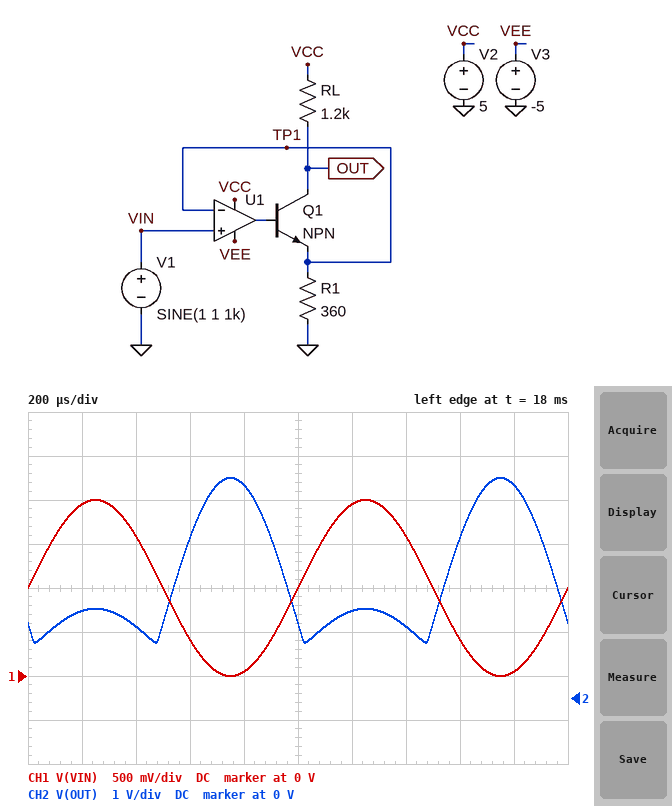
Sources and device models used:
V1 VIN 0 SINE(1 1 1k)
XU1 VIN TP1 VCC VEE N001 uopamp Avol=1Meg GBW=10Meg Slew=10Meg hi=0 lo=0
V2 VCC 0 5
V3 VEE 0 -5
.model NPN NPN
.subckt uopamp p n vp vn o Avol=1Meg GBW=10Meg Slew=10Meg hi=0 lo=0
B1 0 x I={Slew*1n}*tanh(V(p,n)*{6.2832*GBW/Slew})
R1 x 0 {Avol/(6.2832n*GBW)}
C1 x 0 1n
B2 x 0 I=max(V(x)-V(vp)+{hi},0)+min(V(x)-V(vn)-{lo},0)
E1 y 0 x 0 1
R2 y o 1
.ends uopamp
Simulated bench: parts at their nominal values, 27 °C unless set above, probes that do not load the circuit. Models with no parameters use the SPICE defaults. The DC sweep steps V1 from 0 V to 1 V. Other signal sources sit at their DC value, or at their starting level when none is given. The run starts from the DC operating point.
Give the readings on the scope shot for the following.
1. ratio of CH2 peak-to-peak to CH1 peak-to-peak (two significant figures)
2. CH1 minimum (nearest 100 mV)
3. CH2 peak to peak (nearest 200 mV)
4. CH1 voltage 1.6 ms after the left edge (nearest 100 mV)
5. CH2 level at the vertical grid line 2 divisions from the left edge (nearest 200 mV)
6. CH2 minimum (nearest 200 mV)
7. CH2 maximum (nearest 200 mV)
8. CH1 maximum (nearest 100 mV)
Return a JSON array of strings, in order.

["1.9", "0 V", "3.8 V", "400 mV", "1.6 V", "1.2 V", "5.0 V", "2.0 V"]
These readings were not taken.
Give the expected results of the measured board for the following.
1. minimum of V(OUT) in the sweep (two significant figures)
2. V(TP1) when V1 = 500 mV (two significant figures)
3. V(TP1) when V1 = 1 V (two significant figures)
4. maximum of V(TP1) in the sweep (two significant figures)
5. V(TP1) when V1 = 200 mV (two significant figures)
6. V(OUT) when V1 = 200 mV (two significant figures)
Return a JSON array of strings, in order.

["1.7 V", "500 mV", "1.0 V", "1.0 V", "200 mV", "4.3 V"]
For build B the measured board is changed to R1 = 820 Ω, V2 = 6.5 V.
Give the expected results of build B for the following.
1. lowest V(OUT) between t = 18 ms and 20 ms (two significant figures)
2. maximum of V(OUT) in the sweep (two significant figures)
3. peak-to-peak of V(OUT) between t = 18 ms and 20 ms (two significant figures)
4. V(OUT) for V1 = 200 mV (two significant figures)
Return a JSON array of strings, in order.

["3.6 V", "6.5 V", "2.9 V", "6.2 V"]
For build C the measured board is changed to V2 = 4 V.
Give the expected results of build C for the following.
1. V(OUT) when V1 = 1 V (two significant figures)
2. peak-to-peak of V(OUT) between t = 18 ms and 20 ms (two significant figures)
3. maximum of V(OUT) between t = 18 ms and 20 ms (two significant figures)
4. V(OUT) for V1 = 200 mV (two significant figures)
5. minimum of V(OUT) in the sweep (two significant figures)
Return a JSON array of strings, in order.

["1.1 V", "3.0 V", "4.0 V", "3.3 V", "1.0 V"]
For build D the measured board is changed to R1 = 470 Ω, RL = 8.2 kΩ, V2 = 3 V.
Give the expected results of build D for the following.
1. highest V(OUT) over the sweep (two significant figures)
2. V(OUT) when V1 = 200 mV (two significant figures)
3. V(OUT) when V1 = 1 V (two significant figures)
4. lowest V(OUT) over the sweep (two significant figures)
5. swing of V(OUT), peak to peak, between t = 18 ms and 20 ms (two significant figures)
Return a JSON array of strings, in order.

["3.0 V", "250 mV", "1.0 V", "240 mV", "2.8 V"]
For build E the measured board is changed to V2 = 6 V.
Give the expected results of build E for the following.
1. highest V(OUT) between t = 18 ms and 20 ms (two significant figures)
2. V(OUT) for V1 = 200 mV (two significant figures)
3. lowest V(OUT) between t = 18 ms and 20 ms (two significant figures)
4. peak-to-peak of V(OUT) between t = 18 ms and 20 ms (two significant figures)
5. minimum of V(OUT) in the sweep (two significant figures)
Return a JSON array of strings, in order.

["6.0 V", "5.3 V", "1.5 V", "4.5 V", "2.7 V"]
